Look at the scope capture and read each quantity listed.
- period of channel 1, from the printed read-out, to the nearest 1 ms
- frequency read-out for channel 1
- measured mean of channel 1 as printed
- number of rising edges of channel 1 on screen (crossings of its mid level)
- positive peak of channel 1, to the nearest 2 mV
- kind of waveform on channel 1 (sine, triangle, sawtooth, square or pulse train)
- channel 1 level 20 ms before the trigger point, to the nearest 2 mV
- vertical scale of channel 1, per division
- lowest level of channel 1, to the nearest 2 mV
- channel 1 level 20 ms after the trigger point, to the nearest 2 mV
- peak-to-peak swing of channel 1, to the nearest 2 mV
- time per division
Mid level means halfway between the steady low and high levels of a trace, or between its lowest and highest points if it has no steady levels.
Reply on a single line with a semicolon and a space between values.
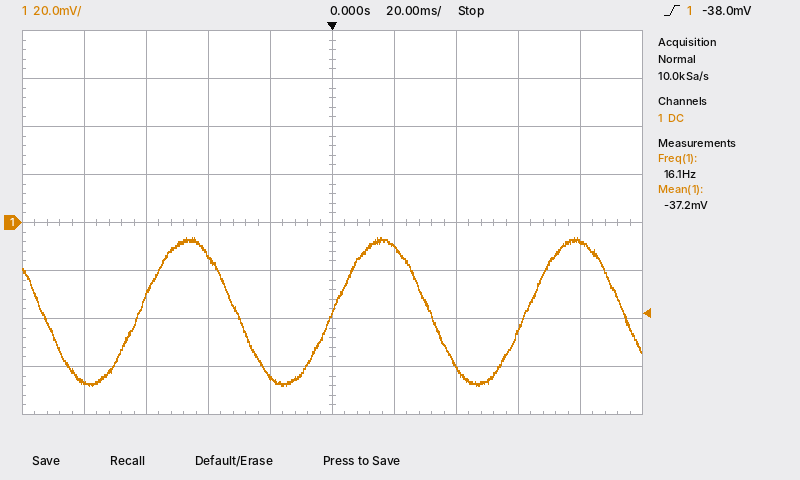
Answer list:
62 ms; 16.1 Hz; -37.2 mV; 3; -6 mV; sine; -64 mV; 20 mV; -68 mV; -10 mV; 62 mV; 20 ms
